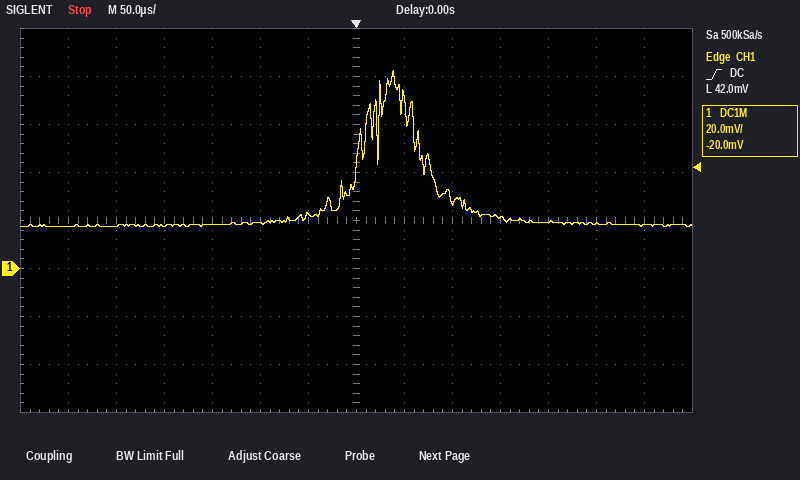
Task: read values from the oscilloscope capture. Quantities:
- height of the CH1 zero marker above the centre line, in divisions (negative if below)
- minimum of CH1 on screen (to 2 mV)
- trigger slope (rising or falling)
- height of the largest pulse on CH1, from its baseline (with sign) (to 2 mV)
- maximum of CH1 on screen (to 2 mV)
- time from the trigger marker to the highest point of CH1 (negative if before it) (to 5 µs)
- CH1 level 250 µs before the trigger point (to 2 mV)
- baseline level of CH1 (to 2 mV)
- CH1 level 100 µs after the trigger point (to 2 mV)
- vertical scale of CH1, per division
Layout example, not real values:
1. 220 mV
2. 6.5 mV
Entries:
1. -1.0 div
2. 18 mV
3. rising
4. +64 mV
5. 82 mV
6. +40 µs
7. 18 mV
8. 18 mV
9. 28 mV
10. 20 mV
